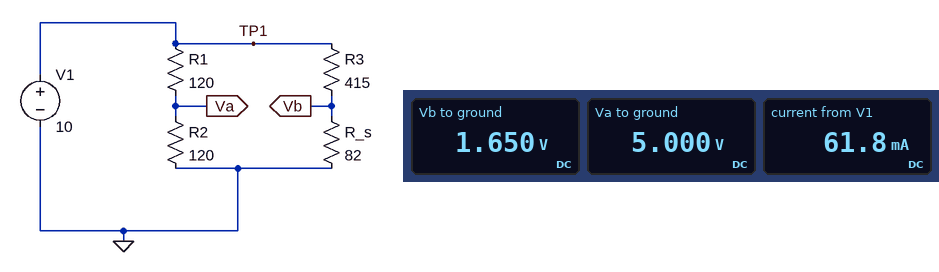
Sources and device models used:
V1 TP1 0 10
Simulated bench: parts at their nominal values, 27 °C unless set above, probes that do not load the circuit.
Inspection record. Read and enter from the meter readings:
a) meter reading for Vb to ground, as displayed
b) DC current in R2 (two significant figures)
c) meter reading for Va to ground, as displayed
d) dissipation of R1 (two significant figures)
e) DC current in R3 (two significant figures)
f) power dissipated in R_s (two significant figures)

1.650 V
42 mA
5.000 V
210 mW
20 mA
33 mW
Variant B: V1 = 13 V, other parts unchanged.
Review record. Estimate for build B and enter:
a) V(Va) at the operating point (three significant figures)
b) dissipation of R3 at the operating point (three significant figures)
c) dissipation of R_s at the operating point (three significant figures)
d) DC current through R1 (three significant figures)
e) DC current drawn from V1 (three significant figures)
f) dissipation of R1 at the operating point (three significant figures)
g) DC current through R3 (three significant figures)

6.50 V
284 mW
56.1 mW
54.2 mA
80.3 mA
352 mW
26.2 mA
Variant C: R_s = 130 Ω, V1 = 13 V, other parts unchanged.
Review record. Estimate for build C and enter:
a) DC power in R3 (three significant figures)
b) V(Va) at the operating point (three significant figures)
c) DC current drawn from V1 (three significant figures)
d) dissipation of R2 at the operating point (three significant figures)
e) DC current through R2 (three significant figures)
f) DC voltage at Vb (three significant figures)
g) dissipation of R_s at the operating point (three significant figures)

236 mW
6.50 V
78.0 mA
352 mW
54.2 mA
3.10 V
74.0 mW
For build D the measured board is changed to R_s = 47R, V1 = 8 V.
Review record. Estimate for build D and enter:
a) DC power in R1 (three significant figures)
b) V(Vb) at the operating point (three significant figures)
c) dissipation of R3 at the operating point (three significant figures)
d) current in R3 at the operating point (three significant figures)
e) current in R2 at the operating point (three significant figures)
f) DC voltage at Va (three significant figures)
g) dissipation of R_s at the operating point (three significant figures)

133 mW
814 mV
124 mW
17.3 mA
33.3 mA
4.00 V
14.1 mW
